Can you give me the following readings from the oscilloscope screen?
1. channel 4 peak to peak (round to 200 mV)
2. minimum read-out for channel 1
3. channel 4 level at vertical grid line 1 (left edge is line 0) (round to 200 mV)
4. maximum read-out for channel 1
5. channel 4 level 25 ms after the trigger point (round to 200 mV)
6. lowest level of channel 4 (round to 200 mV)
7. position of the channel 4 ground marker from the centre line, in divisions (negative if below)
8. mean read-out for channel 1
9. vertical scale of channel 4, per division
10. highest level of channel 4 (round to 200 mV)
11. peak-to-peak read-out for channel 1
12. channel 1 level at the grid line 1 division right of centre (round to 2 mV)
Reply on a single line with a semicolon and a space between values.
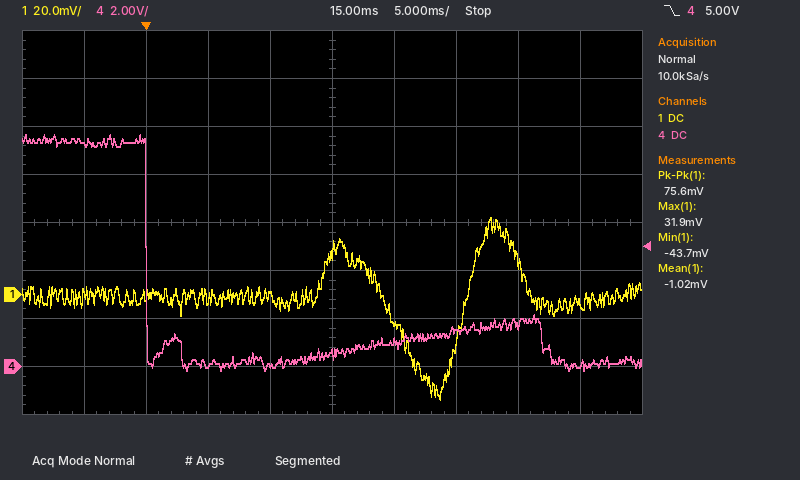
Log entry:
9.8 V; -43.7 mV; 9.2 V; 31.9 mV; 1.4 V; -200 mV; -3.0 div; -1.02 mV; 2 V; 9.6 V; 75.6 mV; -12 mV
